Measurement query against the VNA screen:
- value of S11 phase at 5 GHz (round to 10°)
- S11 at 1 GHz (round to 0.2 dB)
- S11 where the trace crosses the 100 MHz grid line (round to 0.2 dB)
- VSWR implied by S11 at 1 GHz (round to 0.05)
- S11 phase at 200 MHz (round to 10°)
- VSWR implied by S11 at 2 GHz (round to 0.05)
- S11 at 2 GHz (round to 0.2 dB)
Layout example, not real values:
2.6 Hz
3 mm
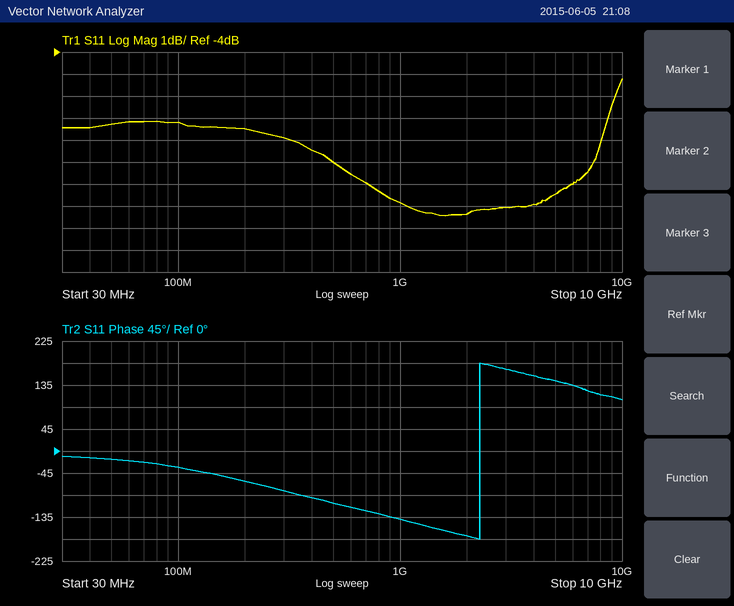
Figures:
140°
-10.8 dB
-7.2 dB
1.80
-60°
1.75
-11.4 dB
